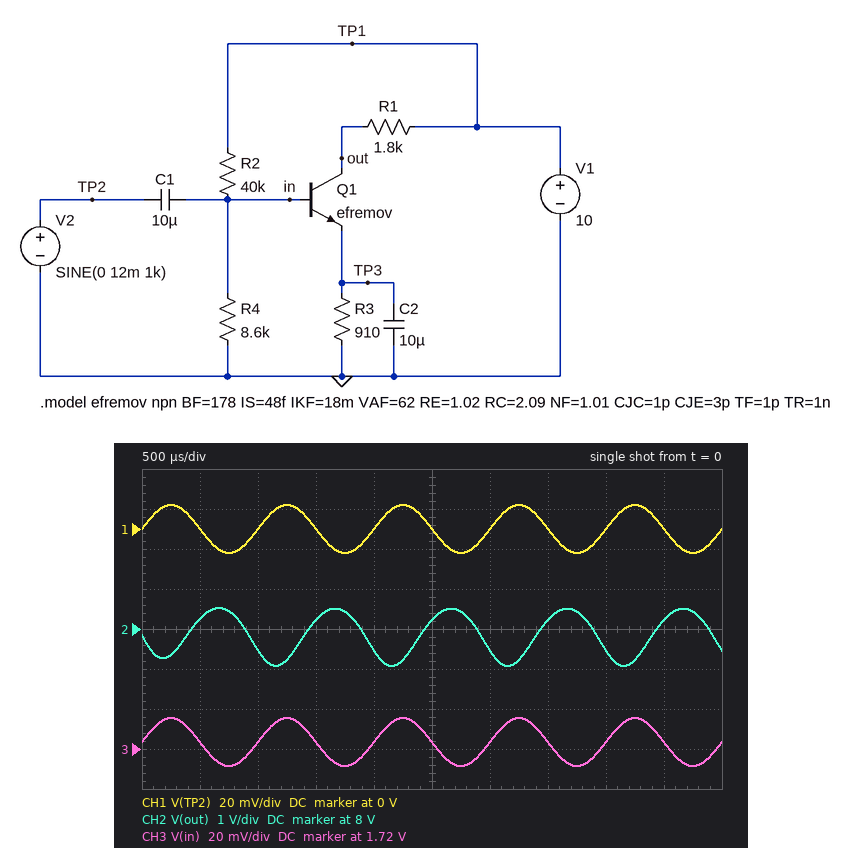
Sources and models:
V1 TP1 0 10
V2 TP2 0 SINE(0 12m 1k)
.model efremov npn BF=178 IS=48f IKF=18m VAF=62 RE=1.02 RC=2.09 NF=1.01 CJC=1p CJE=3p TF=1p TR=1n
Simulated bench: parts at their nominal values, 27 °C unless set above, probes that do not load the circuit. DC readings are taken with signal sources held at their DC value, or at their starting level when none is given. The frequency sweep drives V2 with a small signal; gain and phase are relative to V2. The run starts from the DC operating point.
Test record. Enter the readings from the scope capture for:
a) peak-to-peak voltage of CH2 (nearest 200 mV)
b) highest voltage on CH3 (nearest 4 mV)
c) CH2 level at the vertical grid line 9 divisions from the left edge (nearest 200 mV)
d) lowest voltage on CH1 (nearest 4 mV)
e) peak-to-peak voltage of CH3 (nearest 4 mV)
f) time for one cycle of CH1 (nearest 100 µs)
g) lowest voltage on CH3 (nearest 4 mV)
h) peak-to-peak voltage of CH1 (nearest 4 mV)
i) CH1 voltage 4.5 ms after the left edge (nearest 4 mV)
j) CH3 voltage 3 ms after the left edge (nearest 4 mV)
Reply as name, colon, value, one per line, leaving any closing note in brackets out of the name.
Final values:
peak-to-peak voltage of CH2: 1.4 V
highest voltage on CH3: 1.736 V
CH2 level at the vertical grid line 9 divisions from the left edge: 8.2 V
lowest voltage on CH1: -12 mV
peak-to-peak voltage of CH3: 24 mV
time for one cycle of CH1: 1.0 ms
lowest voltage on CH3: 1.712 V
peak-to-peak voltage of CH1: 24 mV
CH1 voltage 4.5 ms after the left edge: 0 V
CH3 voltage 3 ms after the left edge: 1.724 V
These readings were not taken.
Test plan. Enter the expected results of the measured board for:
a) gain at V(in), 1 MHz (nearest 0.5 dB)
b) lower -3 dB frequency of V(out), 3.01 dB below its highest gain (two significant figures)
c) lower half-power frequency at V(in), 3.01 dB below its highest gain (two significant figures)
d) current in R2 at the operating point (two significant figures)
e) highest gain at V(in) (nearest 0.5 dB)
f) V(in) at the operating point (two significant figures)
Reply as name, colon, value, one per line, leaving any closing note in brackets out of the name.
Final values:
gain at V(in), 1 MHz: 0 dB
lower -3 dB frequency of V(out), 3.01 dB below its highest gain: 670 Hz
lower half-power frequency at V(in), 3.01 dB below its highest gain: 2.4 Hz
current in R2 at the operating point: 210 µA
highest gain at V(in): 0 dB
V(in) at the operating point: 1.7 V
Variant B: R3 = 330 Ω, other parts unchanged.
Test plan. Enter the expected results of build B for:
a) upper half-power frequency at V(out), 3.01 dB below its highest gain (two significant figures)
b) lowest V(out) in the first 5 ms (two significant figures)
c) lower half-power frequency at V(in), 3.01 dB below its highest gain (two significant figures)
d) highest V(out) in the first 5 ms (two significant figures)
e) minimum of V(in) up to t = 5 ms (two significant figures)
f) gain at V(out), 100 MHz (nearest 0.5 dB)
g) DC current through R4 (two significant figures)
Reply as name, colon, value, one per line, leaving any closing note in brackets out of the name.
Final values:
upper half-power frequency at V(out), 3.01 dB below its highest gain: 160 MHz
lowest V(out) in the first 5 ms: 3.6 V
lower half-power frequency at V(in), 3.01 dB below its highest gain: 2.6 Hz
highest V(out) in the first 5 ms: 5.7 V
minimum of V(in) up to t = 5 ms: 1.6 V
gain at V(out), 100 MHz: 42.0 dB
DC current through R4: 190 µA
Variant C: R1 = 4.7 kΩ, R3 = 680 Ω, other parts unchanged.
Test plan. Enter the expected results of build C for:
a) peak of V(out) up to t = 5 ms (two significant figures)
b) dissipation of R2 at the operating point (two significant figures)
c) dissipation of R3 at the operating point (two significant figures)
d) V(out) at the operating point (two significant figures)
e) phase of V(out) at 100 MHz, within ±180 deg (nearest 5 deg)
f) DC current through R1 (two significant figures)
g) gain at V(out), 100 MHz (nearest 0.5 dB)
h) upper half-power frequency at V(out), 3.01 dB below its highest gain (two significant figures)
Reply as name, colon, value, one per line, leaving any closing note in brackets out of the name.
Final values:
peak of V(out) up to t = 5 ms: 4.7 V
dissipation of R2 at the operating point: 1.7 mW
dissipation of R3 at the operating point: 1.7 mW
V(out) at the operating point: 2.7 V
phase of V(out) at 100 MHz, within ±180 deg: 115 deg
DC current through R1: 1.6 mA
gain at V(out), 100 MHz: 40.0 dB
upper half-power frequency at V(out), 3.01 dB below its highest gain: 49 MHz
